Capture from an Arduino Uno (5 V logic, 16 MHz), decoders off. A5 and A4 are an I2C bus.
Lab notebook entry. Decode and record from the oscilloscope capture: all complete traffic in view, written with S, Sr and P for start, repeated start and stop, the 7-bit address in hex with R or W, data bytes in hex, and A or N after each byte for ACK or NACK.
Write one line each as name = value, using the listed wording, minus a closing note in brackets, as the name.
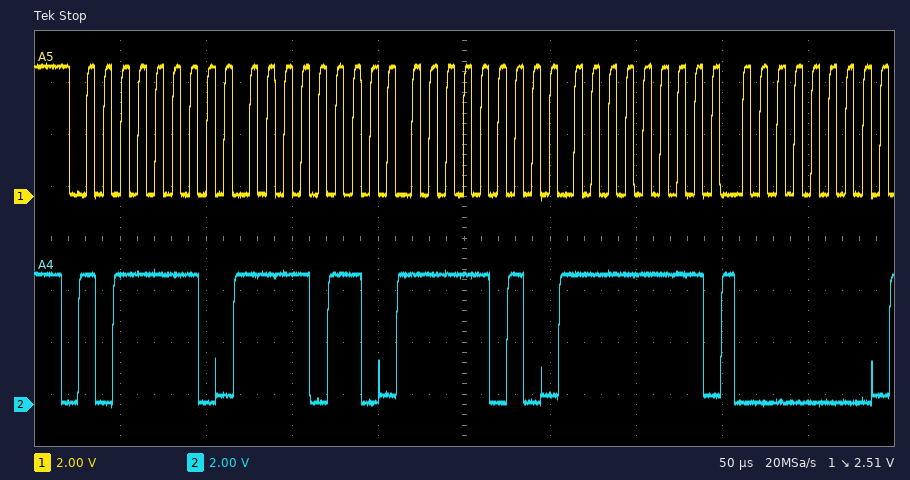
all complete traffic in view, written with S, Sr and P for start, repeated start and stop, the 7-bit address in hex with R or W, data bytes in hex, and A or N after each byte for ACK or NACK = S 5FW A F6 A FA A FF A 00 A
